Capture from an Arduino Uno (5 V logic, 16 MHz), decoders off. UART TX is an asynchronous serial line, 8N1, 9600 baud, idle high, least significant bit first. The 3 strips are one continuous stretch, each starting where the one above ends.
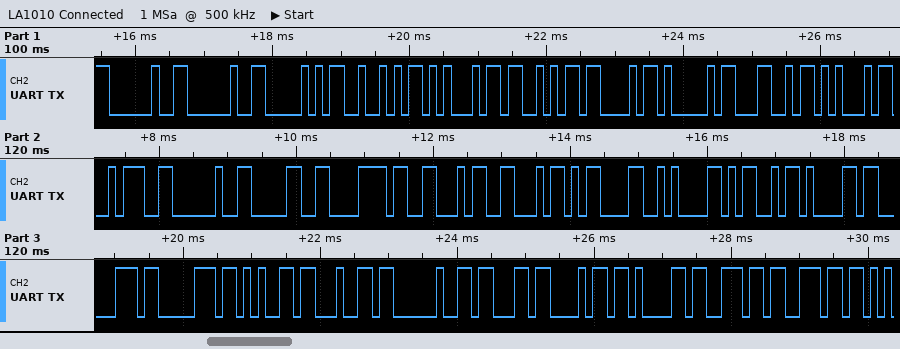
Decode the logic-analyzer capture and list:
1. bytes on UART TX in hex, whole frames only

20 20 50 52 45 53 43 41 4C 45 3A 20 30 78 46 46 0D 0A 4D 61 70 70 65 64 20 63 68 61 6E 6E
